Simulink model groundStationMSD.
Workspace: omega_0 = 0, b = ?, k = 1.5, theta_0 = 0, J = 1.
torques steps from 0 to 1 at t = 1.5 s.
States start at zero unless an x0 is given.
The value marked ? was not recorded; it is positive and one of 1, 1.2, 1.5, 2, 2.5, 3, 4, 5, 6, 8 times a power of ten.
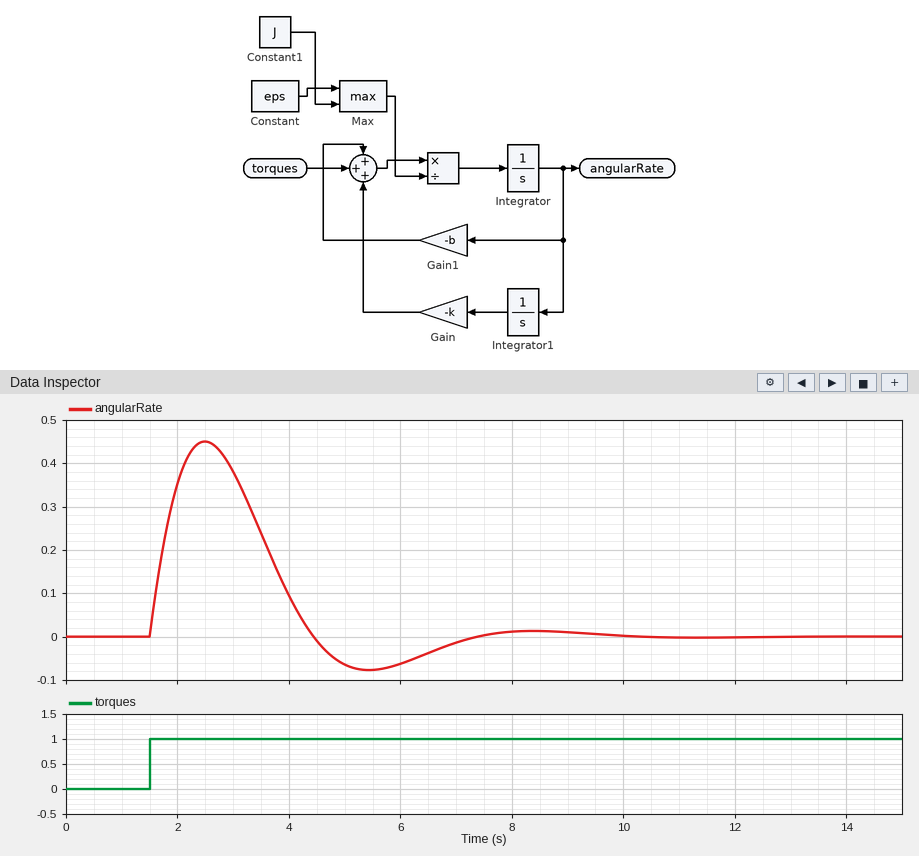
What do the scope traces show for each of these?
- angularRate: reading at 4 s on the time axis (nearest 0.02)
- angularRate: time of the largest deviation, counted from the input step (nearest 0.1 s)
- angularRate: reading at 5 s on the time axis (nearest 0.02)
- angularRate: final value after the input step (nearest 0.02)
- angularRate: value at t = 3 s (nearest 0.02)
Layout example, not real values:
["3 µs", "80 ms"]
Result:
["0.10", "1.0 s", "-0.06", "0.00", "0.38"]
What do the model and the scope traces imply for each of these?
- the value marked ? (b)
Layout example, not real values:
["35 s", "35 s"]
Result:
["1.2"]
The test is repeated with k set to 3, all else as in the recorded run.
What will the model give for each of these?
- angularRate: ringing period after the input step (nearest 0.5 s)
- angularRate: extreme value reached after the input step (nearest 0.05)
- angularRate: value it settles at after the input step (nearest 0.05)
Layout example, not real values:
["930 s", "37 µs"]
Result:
["4.0 s", "0.35", "0.00"]
